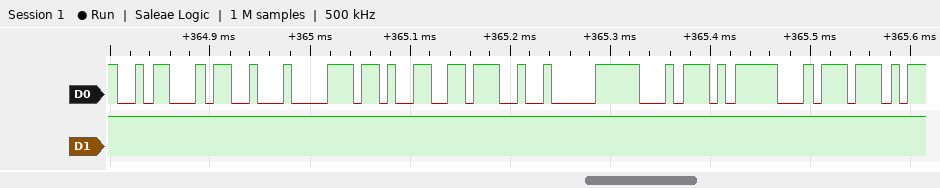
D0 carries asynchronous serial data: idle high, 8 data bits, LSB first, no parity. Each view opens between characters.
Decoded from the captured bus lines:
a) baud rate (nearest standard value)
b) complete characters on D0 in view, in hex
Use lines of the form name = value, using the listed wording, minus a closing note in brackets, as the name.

baud rate = 115200 baud
complete characters on D0 in view, in hex = 1A, 13, B8, 99, 27, F0, 74, 1F, 77
